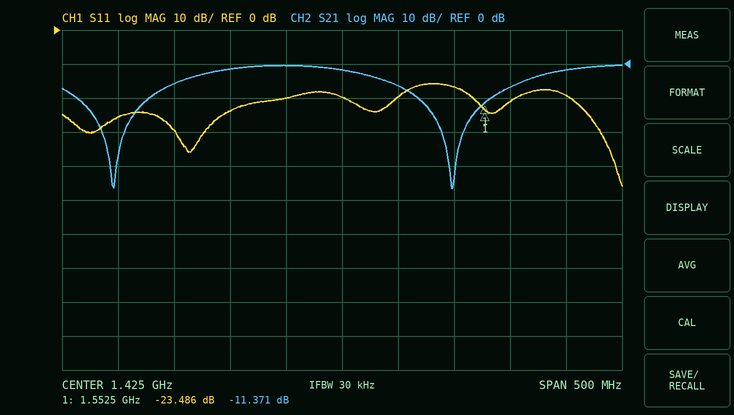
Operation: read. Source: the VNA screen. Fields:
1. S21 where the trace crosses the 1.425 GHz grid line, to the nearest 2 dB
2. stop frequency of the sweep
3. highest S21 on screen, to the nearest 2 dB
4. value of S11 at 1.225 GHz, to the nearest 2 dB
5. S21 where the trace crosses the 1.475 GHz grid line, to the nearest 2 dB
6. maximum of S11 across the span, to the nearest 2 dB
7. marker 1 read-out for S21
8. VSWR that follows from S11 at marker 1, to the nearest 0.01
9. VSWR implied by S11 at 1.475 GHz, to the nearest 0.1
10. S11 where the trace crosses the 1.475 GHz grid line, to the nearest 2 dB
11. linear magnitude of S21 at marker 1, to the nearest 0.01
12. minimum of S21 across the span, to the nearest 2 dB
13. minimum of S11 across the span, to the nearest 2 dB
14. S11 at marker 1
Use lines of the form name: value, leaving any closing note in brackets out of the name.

S21 where the trace crosses the 1.425 GHz grid line, to the nearest 2 dB: -2 dB
stop frequency of the sweep: 1.675 GHz
highest S21 on screen, to the nearest 2 dB: 0 dB
value of S11 at 1.225 GHz, to the nearest 2 dB: -26 dB
S21 where the trace crosses the 1.475 GHz grid line, to the nearest 2 dB: -6 dB
maximum of S11 across the span, to the nearest 2 dB: -16 dB
marker 1 read-out for S21: -11.371 dB
VSWR that follows from S11 at marker 1, to the nearest 0.01: 1.14
VSWR implied by S11 at 1.475 GHz, to the nearest 0.1: 1.2
S11 where the trace crosses the 1.475 GHz grid line, to the nearest 2 dB: -20 dB
linear magnitude of S21 at marker 1, to the nearest 0.01: 0.27
minimum of S21 across the span, to the nearest 2 dB: -36 dB
minimum of S11 across the span, to the nearest 2 dB: -46 dB
S11 at marker 1: -23.486 dB
